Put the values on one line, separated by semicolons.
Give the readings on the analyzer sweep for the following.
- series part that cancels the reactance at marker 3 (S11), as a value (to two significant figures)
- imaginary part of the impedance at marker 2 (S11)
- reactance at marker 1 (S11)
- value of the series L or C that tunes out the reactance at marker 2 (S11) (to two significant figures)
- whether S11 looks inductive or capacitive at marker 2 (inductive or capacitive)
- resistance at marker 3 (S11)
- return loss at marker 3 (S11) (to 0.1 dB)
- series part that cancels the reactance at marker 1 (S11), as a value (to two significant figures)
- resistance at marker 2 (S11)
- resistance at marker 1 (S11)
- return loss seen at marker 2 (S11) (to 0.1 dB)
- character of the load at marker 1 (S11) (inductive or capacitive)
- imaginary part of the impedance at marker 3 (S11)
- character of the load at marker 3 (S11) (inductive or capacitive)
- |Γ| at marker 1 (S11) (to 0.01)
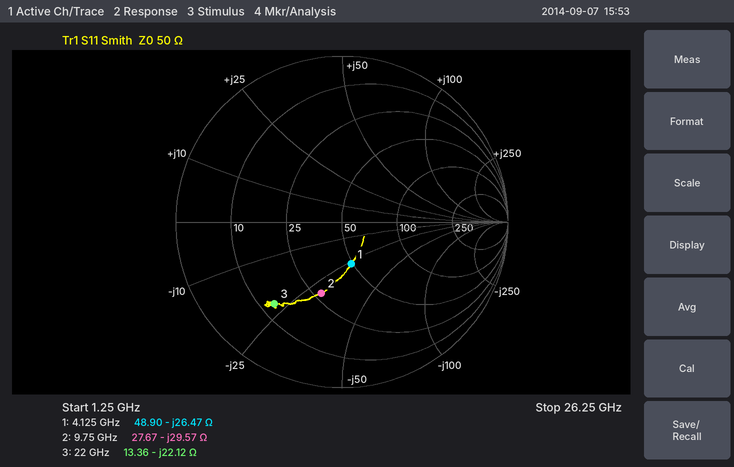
160 pH; -29.57 Ω; -26.47 Ω; 480 pH; capacitive; 13.36 Ω; 3.9 dB; 1.0 nH; 27.67 Ω; 48.90 Ω; 7.0 dB; capacitive; -22.12 Ω; capacitive; 0.26
